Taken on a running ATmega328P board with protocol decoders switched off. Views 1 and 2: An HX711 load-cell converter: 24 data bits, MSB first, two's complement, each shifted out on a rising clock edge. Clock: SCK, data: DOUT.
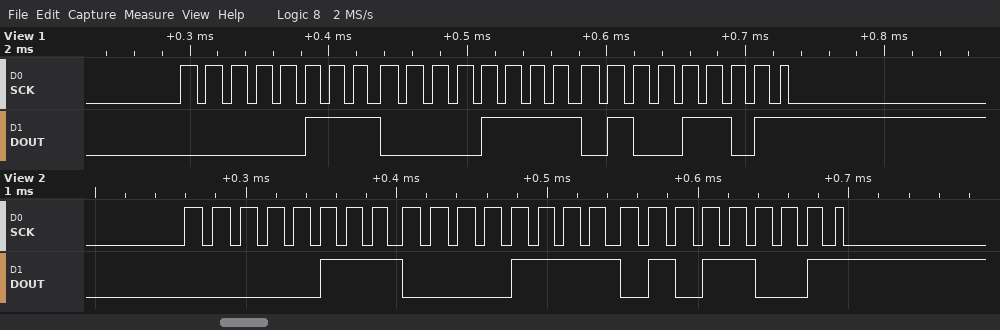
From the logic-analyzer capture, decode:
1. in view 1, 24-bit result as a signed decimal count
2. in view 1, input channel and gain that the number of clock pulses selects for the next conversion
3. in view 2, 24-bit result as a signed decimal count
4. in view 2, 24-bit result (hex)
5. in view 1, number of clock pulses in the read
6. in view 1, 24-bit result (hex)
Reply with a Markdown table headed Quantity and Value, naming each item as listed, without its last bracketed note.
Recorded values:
| Quantity | Value |
|---|---|
| in view 1, 24-bit result as a signed decimal count | 462669 |
| in view 1, input channel and gain that the number of clock pulses selects for the next conversion | channel A, gain 128 |
| in view 2, 24-bit result as a signed decimal count | 462681 |
| in view 2, 24-bit result | 0x070F59 |
| in view 1, number of clock pulses in the read | 25 |
| in view 1, 24-bit result | 0x070F4D |
